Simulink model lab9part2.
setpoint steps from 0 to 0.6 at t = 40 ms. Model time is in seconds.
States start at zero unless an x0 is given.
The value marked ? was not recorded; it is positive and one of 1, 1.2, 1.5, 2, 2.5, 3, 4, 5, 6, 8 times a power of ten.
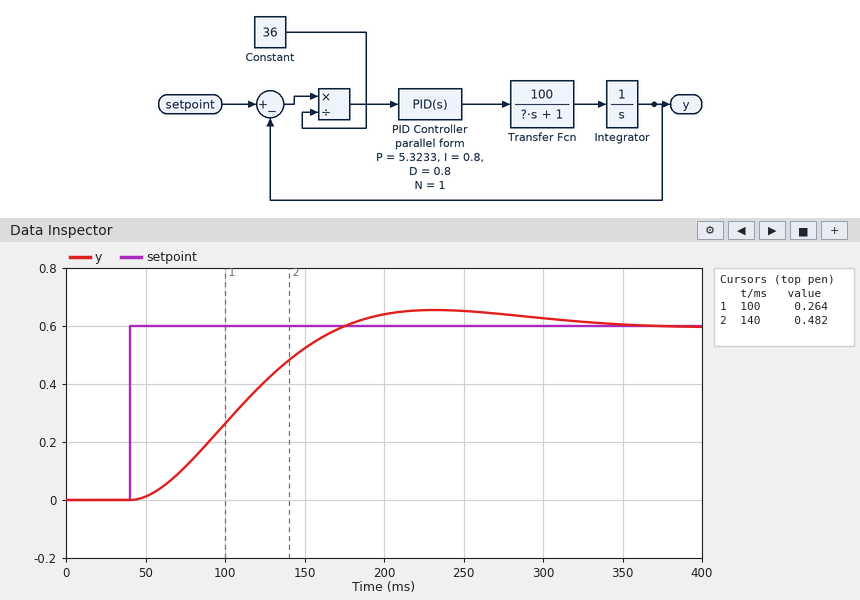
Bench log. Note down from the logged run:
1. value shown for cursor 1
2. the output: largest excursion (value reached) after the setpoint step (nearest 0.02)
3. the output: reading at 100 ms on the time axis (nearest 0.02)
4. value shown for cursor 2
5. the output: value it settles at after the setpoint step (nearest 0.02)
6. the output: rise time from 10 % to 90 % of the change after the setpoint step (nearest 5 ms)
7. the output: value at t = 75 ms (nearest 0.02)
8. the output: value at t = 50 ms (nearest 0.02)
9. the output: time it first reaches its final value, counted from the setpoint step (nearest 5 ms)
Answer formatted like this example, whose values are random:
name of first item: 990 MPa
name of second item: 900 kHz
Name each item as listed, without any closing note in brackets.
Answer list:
value shown for cursor 1: 0.264
the output: largest excursion (value reached) after the setpoint step: 0.66
the output: reading at 100 ms on the time axis: 0.26
value shown for cursor 2: 0.482
the output: value it settles at after the setpoint step: 0.60
the output: rise time from 10 % to 90 % of the change after the setpoint step: 90 ms
the output: value at t = 75 ms: 0.12
the output: value at t = 50 ms: 0.02
the output: time it first reaches its final value, counted from the setpoint step: 135 ms
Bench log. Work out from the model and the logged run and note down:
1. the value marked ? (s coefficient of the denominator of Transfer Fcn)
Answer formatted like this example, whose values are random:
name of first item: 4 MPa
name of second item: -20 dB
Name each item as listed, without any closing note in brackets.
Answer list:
the value marked ?: 0.04
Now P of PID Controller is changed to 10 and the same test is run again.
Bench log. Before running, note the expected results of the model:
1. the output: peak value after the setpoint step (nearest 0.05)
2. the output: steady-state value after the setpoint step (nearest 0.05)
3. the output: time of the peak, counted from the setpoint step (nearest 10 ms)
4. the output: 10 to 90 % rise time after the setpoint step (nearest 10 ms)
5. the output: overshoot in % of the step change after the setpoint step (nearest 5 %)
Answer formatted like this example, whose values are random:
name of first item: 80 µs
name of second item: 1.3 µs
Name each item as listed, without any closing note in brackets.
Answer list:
the output: peak value after the setpoint step: 0.70
the output: steady-state value after the setpoint step: 0.60
the output: time of the peak, counted from the setpoint step: 130 ms
the output: 10 to 90 % rise time after the setpoint step: 60 ms
the output: overshoot in % of the step change after the setpoint step: 20 %
